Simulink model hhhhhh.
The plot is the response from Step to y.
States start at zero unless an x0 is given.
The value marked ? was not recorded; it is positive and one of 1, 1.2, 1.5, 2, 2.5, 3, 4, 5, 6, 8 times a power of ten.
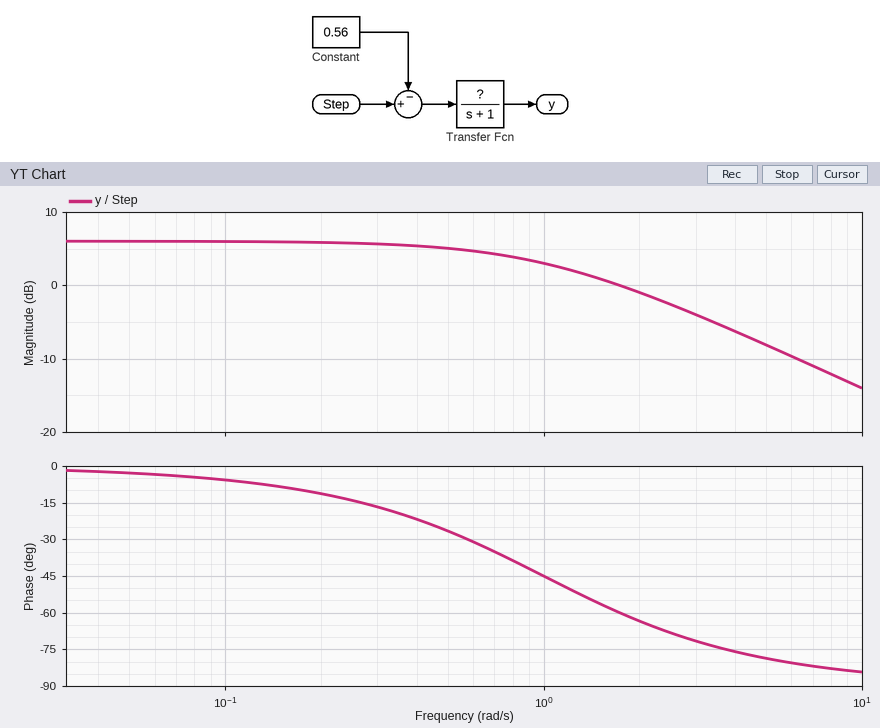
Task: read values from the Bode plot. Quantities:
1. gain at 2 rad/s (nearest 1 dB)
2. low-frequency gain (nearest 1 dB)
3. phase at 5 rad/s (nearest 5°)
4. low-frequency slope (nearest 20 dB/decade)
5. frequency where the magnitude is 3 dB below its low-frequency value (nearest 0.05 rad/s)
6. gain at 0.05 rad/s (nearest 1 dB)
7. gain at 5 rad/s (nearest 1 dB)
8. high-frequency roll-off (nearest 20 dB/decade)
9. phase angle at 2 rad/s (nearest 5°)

-1 dB
6 dB
-80°
0 dB/decade
1.00 rad/s
6 dB
-8 dB
-20 dB/decade
-65°
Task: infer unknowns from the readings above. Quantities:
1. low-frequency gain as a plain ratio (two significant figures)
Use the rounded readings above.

2.0
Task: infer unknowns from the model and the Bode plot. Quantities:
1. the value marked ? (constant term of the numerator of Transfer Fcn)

2
